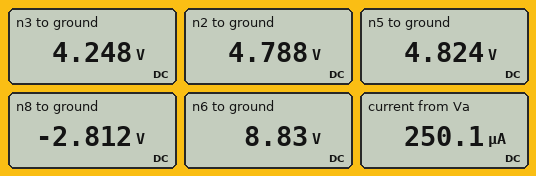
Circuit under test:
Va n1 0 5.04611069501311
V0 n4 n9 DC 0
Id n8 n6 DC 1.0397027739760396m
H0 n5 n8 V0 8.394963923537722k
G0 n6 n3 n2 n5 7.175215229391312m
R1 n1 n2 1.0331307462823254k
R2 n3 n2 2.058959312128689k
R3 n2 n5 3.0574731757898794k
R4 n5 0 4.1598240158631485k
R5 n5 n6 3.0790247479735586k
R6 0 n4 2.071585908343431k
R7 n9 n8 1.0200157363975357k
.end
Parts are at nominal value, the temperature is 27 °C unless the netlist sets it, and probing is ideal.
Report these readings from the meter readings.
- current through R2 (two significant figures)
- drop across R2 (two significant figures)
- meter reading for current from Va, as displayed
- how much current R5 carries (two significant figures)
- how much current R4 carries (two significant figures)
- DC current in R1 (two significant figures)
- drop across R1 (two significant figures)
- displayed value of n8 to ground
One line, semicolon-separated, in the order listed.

260 µA; 540 mV; 250.1 µA; 1.3 mA; 1.2 mA; 250 µA; 260 mV; -2.812 V
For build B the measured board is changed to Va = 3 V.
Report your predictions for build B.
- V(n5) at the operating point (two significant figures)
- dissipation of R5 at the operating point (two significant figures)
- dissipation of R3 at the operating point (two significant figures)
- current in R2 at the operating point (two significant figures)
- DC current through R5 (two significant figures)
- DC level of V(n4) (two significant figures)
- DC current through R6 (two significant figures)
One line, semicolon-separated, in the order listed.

2.9 V; 4.4 mW; 150 nW; 160 µA; 1.2 mA; -1.1 V; 540 µA
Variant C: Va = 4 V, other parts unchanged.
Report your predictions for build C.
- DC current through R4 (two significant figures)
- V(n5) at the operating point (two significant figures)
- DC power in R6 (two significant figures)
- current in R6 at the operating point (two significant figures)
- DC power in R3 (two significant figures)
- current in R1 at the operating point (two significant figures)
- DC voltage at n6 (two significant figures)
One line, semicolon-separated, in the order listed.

920 µA; 3.8 V; 1.1 mW; 720 µA; 270 nW; 200 µA; 7.7 V
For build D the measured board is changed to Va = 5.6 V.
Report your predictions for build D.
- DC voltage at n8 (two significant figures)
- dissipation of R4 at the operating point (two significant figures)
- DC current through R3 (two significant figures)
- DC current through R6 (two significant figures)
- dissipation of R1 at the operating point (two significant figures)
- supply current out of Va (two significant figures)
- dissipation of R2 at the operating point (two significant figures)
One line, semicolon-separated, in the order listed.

-3.1 V; 6.9 mW; 13 µA; 1.0 mA; 80 µW; 280 µA; 170 µW
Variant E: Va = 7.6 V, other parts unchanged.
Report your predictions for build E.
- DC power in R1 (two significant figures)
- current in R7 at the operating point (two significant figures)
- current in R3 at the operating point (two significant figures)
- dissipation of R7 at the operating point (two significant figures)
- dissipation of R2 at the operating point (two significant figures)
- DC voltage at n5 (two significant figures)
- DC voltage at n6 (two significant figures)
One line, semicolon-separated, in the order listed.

150 µW; 1.4 mA; 18 µA; 1.9 mW; 320 µW; 7.3 V; 12 V
